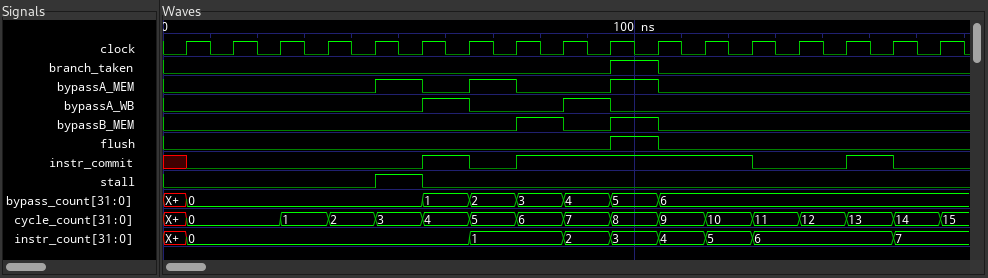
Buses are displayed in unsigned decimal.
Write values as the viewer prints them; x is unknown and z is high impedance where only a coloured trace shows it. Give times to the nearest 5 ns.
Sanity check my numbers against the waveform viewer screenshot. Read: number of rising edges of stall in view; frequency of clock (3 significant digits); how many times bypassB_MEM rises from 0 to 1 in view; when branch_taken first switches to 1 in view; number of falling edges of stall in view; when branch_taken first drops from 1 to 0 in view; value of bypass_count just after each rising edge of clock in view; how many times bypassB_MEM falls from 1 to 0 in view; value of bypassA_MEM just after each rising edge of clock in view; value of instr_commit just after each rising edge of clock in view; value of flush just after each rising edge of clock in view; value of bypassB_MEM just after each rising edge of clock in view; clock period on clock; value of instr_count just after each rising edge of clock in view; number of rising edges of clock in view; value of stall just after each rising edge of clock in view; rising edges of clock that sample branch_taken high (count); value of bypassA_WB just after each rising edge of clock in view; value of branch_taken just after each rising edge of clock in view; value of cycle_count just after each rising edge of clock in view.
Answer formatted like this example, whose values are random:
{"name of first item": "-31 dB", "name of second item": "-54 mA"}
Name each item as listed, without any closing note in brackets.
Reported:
{"number of rising edges of stall in view": "1", "frequency of clock": "100 MHz", "how many times bypassB_MEM rises from 0 to 1 in view": "2", "when branch_taken first switches to 1 in view": "95 ns", "number of falling edges of stall in view": "1", "when branch_taken first drops from 1 to 0 in view": "105 ns", "value of bypass_count just after each rising edge of clock in view": "0, 0, 0, 0, 0, 1, 2, 3, 4, 5, 6, 6, 6, 6, 6, 6, 6", "how many times bypassB_MEM falls from 1 to 0 in view": "2", "value of bypassA_MEM just after each rising edge of clock in view": "0 0 0 0 1 0 1 0 0 1 0 0 0 0 0 0 0", "value of instr_commit just after each rising edge of clock in view": "0 0 0 0 0 1 0 1 1 1 1 1 0 0 1 0 0", "value of flush just after each rising edge of clock in view": "0 0 0 0 0 0 0 0 0 1 0 0 0 0 0 0 0", "value of bypassB_MEM just after each rising edge of clock in view": "0 0 0 0 0 0 0 1 0 1 0 0 0 0 0 0 0", "clock period on clock": "10 ns", "value of instr_count just after each rising edge of clock in view": "0, 0, 0, 0, 0, 0, 1, 1, 2, 3, 4, 5, 6, 6, 6, 7, 7", "number of rising edges of clock in view": "17", "value of stall just after each rising edge of clock in view": "0 0 0 0 1 0 0 0 0 0 0 0 0 0 0 0 0", "rising edges of clock that sample branch_taken high": "1", "value of bypassA_WB just after each rising edge of clock in view": "0 0 0 0 0 1 0 0 1 0 0 0 0 0 0 0 0", "value of branch_taken just after each rising edge of clock in view": "0 0 0 0 0 0 0 0 0 1 0 0 0 0 0 0 0", "value of cycle_count just after each rising edge of clock in view": "0, 0, 1, 2, 3, 4, 5, 6, 7, 8, 9, 10, 11, 12, 13, 14, 15"}
